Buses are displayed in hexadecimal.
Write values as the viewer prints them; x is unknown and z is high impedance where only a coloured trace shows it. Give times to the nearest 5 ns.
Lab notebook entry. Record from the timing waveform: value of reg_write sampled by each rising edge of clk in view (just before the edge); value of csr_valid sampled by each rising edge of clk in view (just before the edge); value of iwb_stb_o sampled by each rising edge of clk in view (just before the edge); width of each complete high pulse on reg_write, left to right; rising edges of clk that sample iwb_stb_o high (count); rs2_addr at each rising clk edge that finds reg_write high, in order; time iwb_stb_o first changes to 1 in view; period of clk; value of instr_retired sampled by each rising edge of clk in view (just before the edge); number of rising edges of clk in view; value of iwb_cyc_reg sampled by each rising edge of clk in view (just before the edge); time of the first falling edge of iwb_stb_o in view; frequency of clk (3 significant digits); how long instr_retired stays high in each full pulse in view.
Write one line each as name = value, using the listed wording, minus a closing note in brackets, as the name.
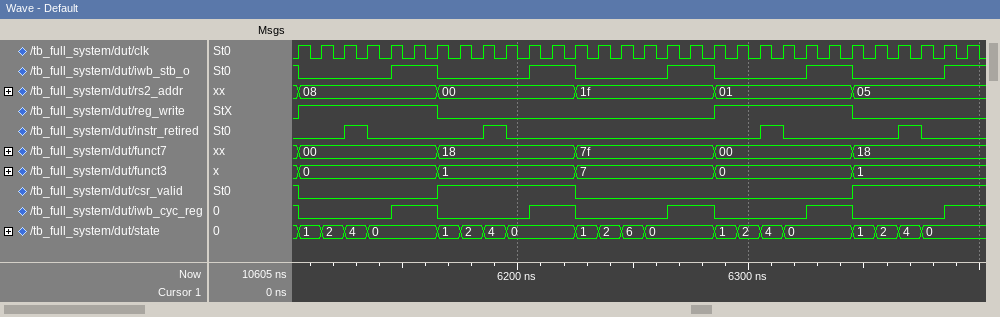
value of reg_write sampled by each rising edge of clk in view = 0 1 1 1 1 1 1 0 0 0 0 0 0 0 0 0 0 0 0 1 1 1 1 1 1 0 0 0 0 0
value of csr_valid sampled by each rising edge of clk in view = 1 0 0 0 0 0 0 1 1 1 1 1 1 0 0 0 0 0 0 0 0 0 0 0 0 1 1 1 1 1
value of iwb_stb_o sampled by each rising edge of clk in view = 1 0 0 0 0 1 1 0 0 0 0 1 1 0 0 0 0 1 1 0 0 0 0 1 1 0 0 0 0 1
width of each complete high pulse on reg_write, left to right = 60 ns, 60 ns
rising edges of clk that sample iwb_stb_o high = 10
rs2_addr at each rising clk edge that finds reg_write high, in order = 08, 08, 08, 08, 08, 08, 01, 01, 01, 01, 01, 01
time iwb_stb_o first changes to 1 in view = 6145 ns
period of clk = 10 ns
value of instr_retired sampled by each rising edge of clk in view = 0 0 0 1 0 0 0 0 0 1 0 0 0 0 0 0 0 0 0 0 0 1 0 0 0 0 0 1 0 0
number of rising edges of clk in view = 30
value of iwb_cyc_reg sampled by each rising edge of clk in view = 1 0 0 0 0 1 1 0 0 0 0 1 1 0 0 0 0 1 1 0 0 0 0 1 1 0 0 0 0 1
time of the first falling edge of iwb_stb_o in view = 6105 ns
frequency of clk = 100 MHz
how long instr_retired stays high in each full pulse in view = 10 ns, 10 ns, 10 ns, 10 ns
